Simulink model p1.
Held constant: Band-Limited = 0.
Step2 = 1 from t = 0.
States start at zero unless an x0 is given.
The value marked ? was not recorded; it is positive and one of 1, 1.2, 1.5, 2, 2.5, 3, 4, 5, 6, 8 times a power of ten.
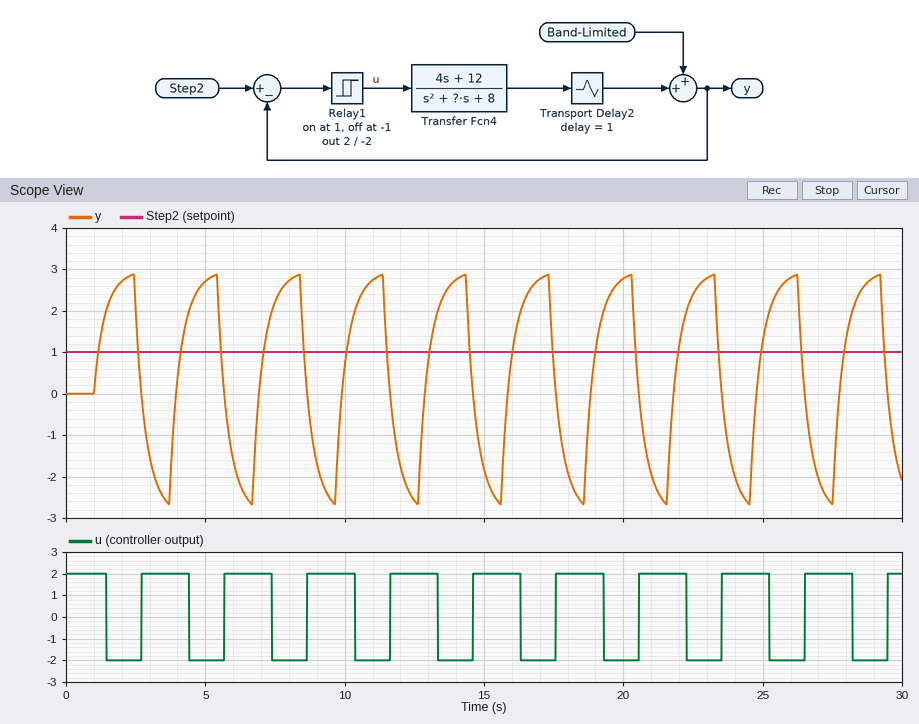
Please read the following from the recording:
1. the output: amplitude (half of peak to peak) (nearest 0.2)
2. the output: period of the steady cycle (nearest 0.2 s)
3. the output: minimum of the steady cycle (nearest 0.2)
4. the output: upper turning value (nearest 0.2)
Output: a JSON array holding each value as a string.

["2.8", "3.0 s", "-2.6", "2.8"]
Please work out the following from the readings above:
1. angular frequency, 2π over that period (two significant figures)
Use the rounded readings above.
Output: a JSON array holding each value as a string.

["2.1 rad/s"]
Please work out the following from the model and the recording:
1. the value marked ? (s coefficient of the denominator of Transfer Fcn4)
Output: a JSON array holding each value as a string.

["6"]
